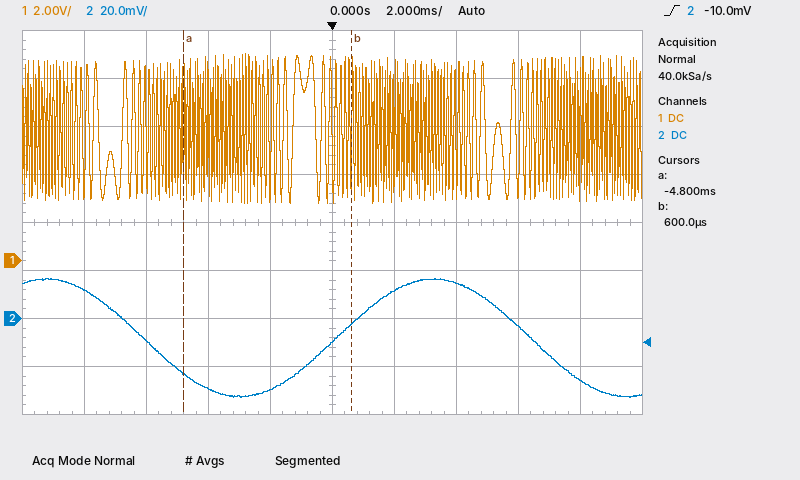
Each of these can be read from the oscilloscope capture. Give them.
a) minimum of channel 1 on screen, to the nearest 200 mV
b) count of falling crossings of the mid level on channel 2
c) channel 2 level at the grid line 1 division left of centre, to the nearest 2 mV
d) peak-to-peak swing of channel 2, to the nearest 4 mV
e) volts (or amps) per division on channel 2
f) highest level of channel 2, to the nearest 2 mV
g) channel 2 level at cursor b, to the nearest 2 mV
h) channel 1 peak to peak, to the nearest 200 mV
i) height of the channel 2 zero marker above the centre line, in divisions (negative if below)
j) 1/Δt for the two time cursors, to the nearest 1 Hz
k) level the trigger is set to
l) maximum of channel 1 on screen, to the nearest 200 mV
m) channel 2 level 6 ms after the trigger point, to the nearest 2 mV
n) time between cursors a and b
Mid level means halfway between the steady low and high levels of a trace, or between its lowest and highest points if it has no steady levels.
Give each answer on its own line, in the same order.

2.4 V
2
-30 mV
48 mV
20 mV
16 mV
-2 mV
6.2 V
-2.0 div
185 Hz
-10.0 mV
8.6 V
-4 mV
5.4 ms
